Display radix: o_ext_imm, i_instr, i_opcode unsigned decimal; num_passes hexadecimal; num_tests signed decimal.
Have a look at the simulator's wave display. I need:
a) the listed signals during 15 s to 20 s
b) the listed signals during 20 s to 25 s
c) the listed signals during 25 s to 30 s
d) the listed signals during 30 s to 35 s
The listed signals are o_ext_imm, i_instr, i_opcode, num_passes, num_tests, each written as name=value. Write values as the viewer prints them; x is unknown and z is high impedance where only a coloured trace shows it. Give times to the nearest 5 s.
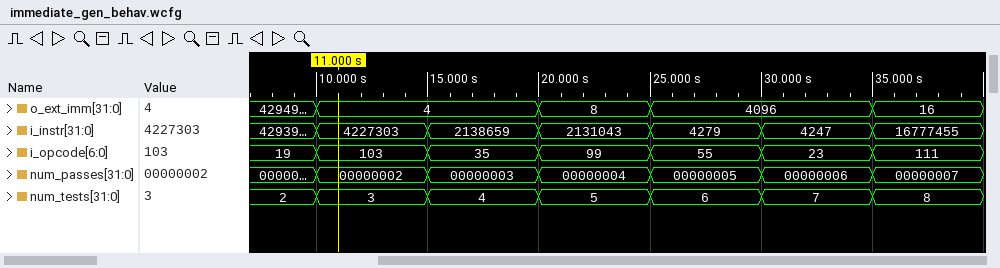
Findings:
o_ext_imm=4, i_instr=2138659, i_opcode=35, num_passes=00000003, num_tests=4
o_ext_imm=8, i_instr=2131043, i_opcode=99, num_passes=00000004, num_tests=5
o_ext_imm=4096, i_instr=4279, i_opcode=55, num_passes=00000005, num_tests=6
o_ext_imm=4096, i_instr=4247, i_opcode=23, num_passes=00000006, num_tests=7
